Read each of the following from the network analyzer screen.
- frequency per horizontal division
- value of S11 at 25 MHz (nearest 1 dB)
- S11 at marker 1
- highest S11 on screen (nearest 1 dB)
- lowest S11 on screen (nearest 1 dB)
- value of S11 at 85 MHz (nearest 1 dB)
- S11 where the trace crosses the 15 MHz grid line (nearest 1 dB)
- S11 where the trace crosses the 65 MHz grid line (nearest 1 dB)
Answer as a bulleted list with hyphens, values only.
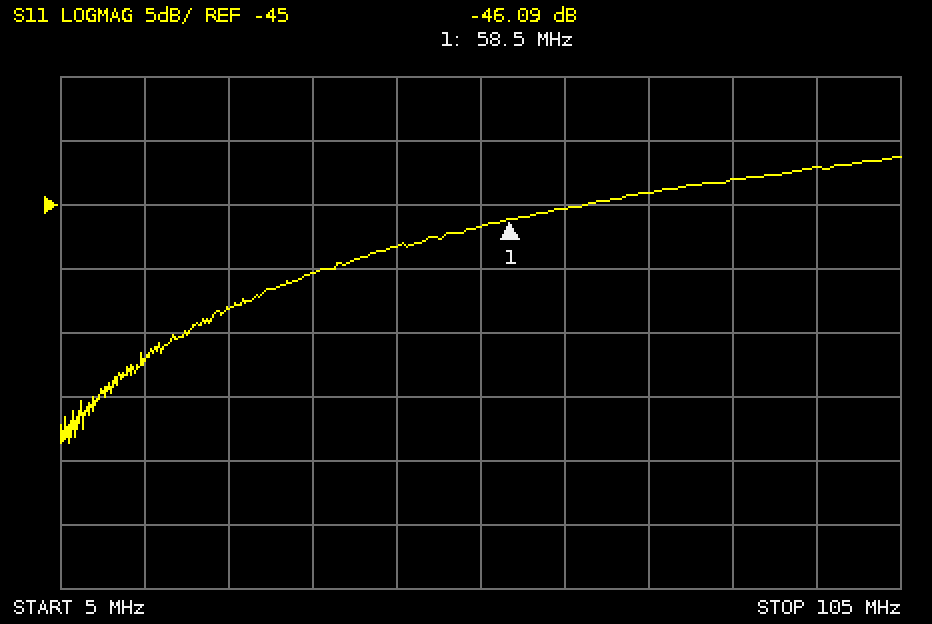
- 10 MHz
- -53 dB
- -46.09 dB
- -41 dB
- -64 dB
- -43 dB
- -57 dB
- -45 dB
